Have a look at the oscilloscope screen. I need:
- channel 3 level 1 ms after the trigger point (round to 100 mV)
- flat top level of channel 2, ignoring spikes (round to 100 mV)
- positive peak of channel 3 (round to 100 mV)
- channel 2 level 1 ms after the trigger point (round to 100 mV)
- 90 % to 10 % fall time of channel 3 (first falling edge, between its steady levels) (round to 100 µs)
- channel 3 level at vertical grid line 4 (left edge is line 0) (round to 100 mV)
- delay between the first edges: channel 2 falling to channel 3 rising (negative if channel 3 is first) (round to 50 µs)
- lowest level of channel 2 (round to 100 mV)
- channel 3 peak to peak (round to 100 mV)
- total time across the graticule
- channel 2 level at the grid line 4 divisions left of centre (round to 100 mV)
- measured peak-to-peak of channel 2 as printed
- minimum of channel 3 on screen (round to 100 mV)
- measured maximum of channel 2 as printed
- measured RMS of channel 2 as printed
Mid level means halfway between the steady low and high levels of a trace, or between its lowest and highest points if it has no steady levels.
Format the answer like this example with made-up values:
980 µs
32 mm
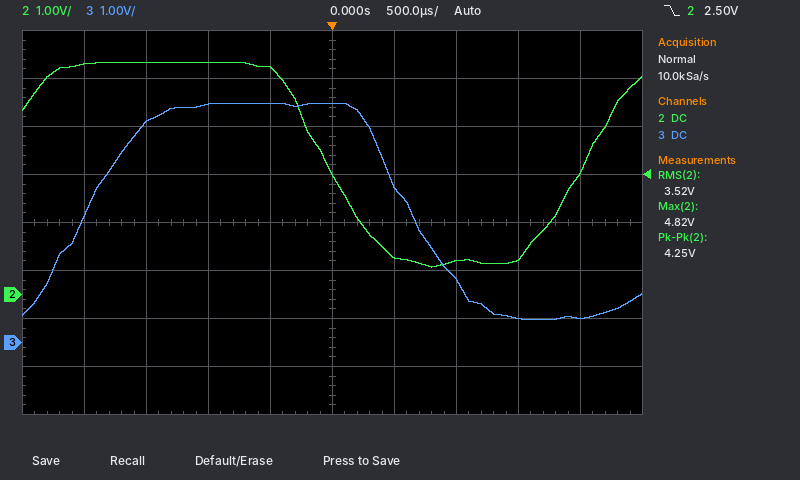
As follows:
1.3 V
4.8 V
5.0 V
700 mV
800 µs
5.0 V
-1.95 ms
600 mV
4.5 V
5 ms
4.8 V
4.25 V
500 mV
4.82 V
3.52 V
